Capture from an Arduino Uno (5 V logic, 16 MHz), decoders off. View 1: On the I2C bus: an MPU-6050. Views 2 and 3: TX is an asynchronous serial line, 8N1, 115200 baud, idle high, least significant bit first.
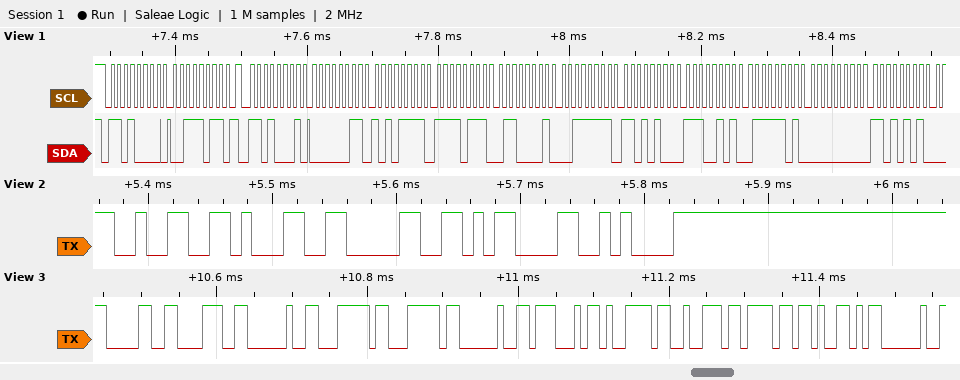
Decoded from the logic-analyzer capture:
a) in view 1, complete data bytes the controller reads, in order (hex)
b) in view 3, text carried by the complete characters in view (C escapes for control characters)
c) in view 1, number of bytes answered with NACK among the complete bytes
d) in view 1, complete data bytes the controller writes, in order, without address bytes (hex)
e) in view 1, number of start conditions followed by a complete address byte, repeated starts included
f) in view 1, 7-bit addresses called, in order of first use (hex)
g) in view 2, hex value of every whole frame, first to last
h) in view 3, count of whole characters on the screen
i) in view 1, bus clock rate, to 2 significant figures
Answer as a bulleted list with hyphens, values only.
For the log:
- 03 AF F7 61 3F D4 E5 7D 00 D5
- "08 || GyroY "
- 0
- 3B
- 2
- 0x68
- 32 31 30 0D 0A
- 12
- 100 kHz
